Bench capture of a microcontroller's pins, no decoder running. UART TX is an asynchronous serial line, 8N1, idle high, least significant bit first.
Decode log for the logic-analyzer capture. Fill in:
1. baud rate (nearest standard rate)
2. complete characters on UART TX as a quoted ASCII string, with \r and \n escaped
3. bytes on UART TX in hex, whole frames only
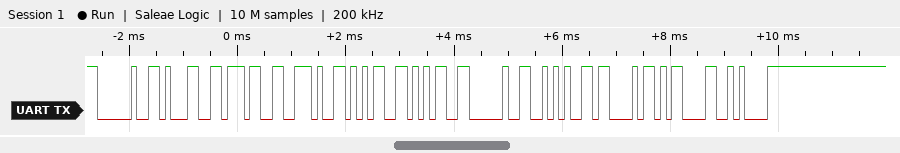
9600 baud
" 17.55 *C\r\n"
0x20 0x31 0x37 0x2E 0x35 0x35 0x20 0x2A 0x43 0x0D 0x0A
